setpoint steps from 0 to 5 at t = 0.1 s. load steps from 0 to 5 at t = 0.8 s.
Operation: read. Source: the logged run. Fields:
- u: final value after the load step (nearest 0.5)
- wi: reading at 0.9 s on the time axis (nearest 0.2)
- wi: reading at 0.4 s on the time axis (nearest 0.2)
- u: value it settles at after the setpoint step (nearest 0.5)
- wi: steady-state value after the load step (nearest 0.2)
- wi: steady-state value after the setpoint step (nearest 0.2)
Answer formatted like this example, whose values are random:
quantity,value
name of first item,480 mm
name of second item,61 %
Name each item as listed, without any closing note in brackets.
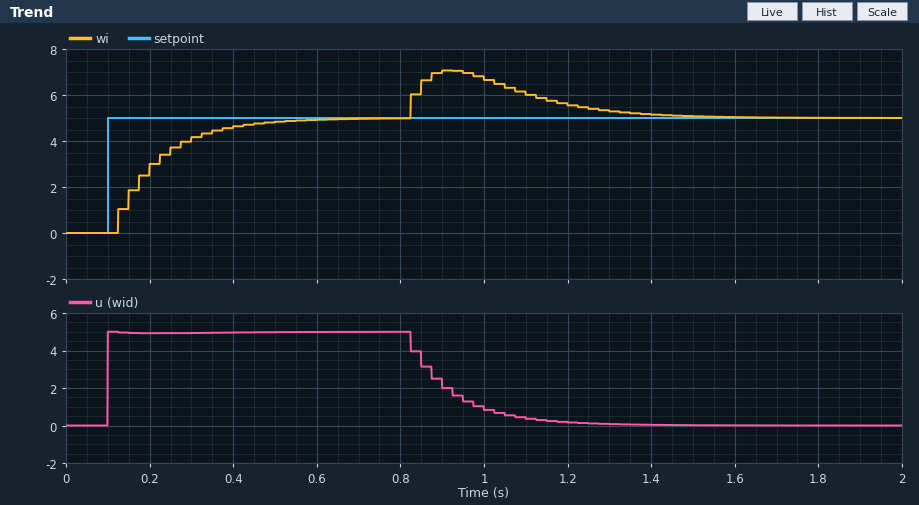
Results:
quantity,value
u: final value after the load step,0.0
wi: reading at 0.9 s on the time axis,7.0
wi: reading at 0.4 s on the time axis,4.6
u: value it settles at after the setpoint step,5.0
wi: steady-state value after the load step,5.0
wi: steady-state value after the setpoint step,5.0
